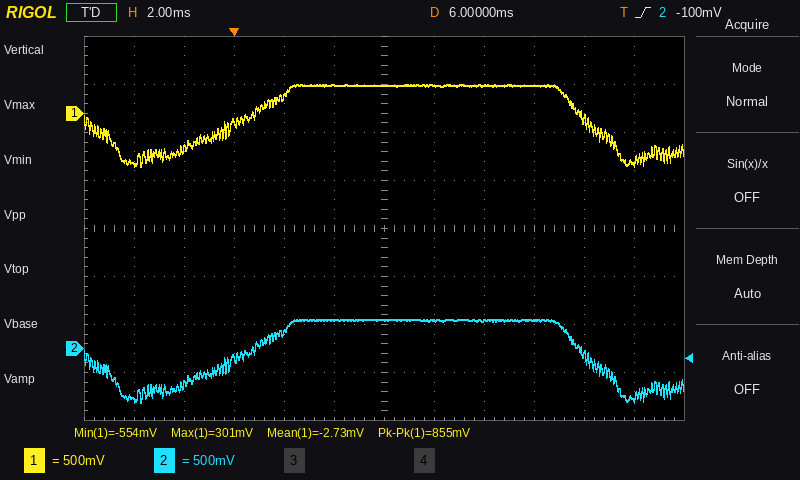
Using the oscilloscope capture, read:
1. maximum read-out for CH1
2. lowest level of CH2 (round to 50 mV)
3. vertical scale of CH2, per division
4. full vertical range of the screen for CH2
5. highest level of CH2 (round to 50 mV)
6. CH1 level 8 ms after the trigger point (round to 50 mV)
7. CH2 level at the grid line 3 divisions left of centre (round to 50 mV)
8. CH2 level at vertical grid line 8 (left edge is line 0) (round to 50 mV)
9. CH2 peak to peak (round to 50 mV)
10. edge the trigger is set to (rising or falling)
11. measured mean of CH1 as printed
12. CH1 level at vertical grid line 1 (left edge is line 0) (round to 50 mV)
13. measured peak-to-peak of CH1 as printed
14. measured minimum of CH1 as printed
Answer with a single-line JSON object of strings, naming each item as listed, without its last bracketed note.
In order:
{"maximum read-out for CH1": "301 mV", "lowest level of CH2": "-550 mV", "vertical scale of CH2, per division": "500 mV", "full vertical range of the screen for CH2": "4 V", "highest level of CH2": "300 mV", "CH1 level 8 ms after the trigger point": "300 mV", "CH2 level at the grid line 3 divisions left of centre": "-100 mV", "CH2 level at vertical grid line 8 (left edge is line 0)": "300 mV", "CH2 peak to peak": "850 mV", "edge the trigger is set to": "rising", "measured mean of CH1 as printed": "-2.73 mV", "CH1 level at vertical grid line 1 (left edge is line 0)": "-550 mV", "measured peak-to-peak of CH1 as printed": "855 mV", "measured minimum of CH1 as printed": "-554 mV"}
